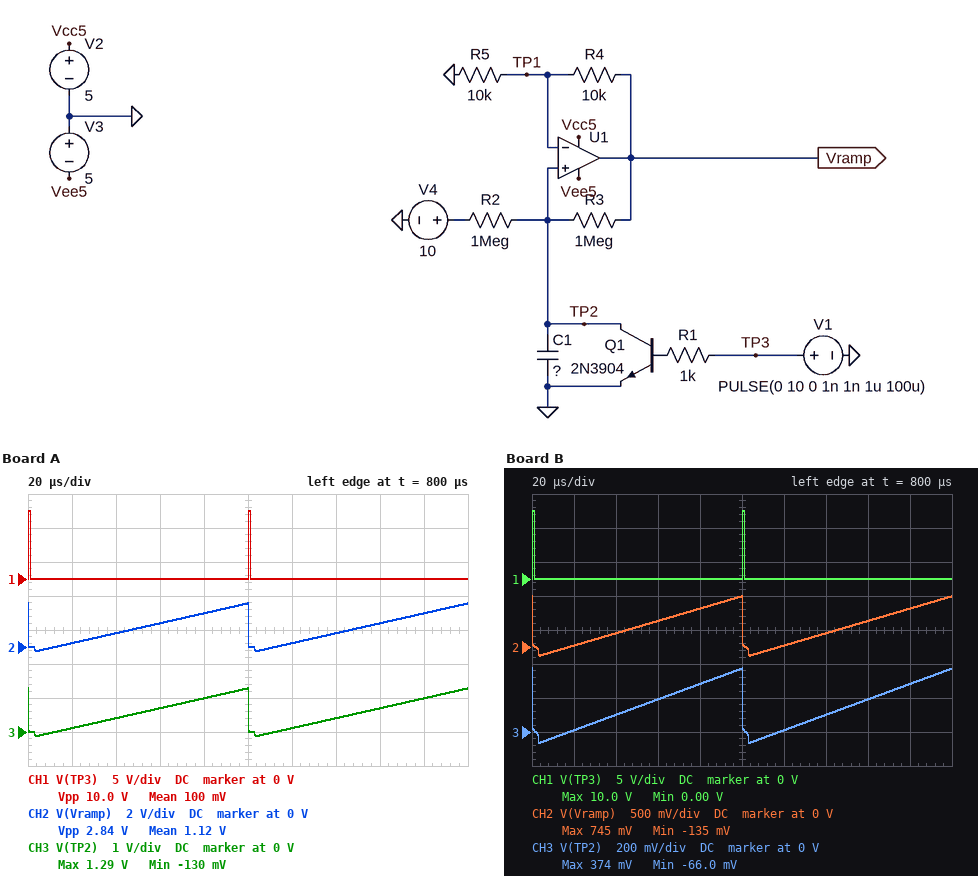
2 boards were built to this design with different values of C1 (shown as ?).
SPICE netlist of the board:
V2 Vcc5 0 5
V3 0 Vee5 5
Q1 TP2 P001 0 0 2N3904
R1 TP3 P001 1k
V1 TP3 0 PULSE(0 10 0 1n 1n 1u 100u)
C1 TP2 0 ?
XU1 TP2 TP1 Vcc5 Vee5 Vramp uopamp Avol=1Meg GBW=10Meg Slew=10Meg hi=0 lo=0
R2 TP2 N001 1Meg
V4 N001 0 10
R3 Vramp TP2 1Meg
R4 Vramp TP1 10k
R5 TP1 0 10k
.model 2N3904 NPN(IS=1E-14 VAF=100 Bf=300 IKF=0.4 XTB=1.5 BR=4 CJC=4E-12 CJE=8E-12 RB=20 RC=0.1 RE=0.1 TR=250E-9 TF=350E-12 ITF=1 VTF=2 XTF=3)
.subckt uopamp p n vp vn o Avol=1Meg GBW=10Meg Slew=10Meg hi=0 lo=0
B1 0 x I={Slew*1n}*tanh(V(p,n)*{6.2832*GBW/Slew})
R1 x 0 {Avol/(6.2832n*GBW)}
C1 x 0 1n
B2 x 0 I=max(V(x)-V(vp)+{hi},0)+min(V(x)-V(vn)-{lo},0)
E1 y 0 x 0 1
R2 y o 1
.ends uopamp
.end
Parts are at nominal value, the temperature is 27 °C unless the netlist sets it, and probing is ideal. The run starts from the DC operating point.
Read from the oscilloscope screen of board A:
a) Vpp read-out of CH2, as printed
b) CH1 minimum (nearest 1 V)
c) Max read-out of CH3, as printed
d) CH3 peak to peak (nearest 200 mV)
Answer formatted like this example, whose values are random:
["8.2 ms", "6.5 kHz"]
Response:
["2.84 V", "0 V", "1.29 V", "1.4 V"]
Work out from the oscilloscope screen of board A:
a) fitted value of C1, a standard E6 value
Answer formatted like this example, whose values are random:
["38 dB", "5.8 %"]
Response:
["680 pF"]
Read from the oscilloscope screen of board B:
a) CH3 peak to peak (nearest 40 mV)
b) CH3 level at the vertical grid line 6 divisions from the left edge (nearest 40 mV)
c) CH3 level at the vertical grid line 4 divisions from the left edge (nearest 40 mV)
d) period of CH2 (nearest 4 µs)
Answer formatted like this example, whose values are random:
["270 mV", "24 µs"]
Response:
["440 mV", "0 V", "280 mV", "100 µs"]
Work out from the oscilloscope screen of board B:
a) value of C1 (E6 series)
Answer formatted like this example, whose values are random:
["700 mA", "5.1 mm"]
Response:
["2.2 nF"]
